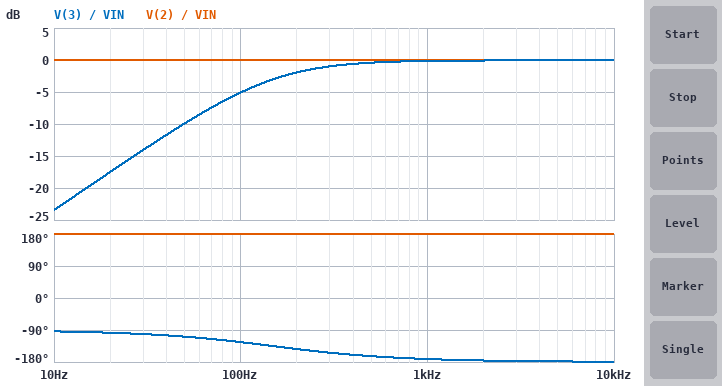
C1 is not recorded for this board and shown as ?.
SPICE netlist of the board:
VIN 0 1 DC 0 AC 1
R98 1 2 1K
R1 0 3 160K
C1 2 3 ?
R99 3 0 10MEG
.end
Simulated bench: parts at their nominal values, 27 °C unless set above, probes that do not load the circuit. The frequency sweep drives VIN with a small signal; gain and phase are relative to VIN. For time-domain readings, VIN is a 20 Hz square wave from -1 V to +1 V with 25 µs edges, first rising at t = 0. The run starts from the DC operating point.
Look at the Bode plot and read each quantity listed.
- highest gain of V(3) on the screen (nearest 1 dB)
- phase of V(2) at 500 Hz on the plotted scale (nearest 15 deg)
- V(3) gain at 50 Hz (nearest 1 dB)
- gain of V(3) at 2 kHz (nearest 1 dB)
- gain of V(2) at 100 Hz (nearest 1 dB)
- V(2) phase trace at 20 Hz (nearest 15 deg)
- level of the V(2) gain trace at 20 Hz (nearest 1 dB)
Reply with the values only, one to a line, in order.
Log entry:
0 dB
180 deg
-10 dB
0 dB
0 dB
180 deg
0 dB
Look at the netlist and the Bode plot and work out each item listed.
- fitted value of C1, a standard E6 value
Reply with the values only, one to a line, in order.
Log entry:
6.8 nF
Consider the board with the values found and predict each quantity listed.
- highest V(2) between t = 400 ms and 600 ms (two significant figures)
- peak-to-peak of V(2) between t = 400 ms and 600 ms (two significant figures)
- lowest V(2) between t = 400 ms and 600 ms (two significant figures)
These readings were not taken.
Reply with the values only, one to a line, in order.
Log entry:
1.0 V
2.0 V
-1.0 V
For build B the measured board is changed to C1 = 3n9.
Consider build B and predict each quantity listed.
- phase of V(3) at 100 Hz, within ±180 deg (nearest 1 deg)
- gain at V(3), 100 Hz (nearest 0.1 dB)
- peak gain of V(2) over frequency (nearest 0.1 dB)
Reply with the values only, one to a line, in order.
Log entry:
-111 deg
-8.9 dB
0 dB
